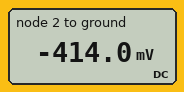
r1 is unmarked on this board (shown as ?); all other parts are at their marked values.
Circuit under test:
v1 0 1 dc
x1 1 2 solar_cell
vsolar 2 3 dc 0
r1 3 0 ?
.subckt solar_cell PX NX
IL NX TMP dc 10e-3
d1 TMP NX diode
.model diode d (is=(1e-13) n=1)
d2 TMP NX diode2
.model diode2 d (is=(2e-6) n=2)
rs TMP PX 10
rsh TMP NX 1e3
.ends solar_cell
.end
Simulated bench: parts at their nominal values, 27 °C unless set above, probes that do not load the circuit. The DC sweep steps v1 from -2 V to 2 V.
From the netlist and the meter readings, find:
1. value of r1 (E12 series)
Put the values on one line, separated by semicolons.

270 Ω
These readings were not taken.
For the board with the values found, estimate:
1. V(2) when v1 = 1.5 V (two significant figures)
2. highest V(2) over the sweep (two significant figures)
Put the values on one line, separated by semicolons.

-1.8 V; 1.5 V
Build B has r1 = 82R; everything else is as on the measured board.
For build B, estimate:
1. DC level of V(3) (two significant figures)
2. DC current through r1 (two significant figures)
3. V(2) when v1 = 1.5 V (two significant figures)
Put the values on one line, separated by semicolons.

-360 mV; 4.4 mA; -860 mV
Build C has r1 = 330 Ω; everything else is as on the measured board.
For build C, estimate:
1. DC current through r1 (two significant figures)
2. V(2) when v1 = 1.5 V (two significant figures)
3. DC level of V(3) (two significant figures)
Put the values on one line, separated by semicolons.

1.3 mA; -1.8 V; -420 mV
